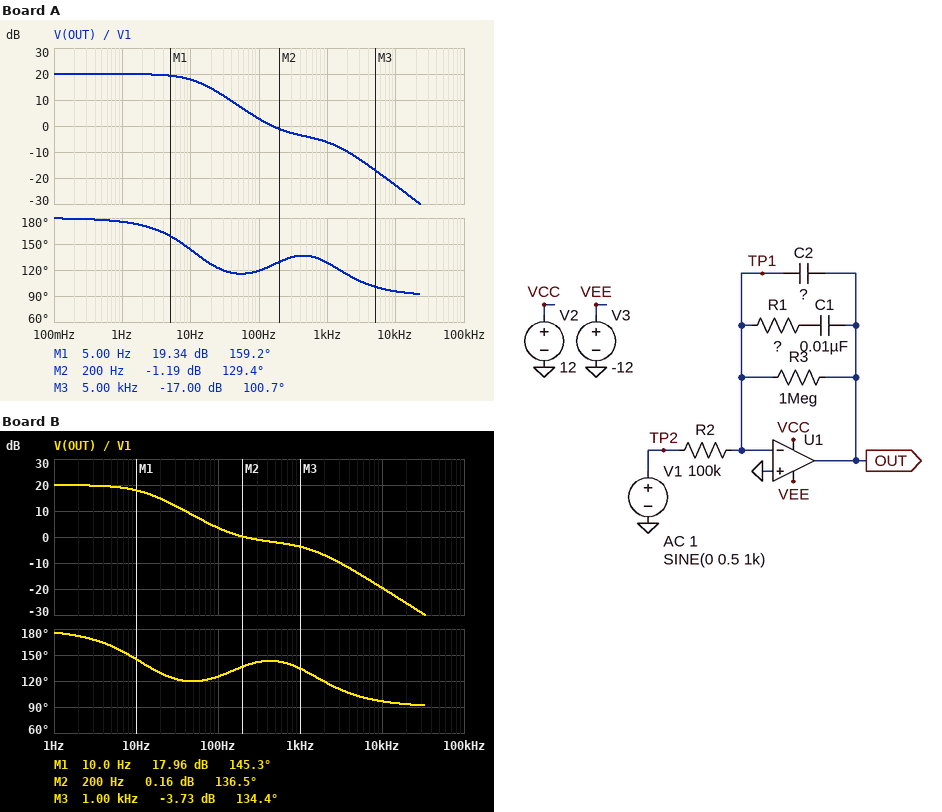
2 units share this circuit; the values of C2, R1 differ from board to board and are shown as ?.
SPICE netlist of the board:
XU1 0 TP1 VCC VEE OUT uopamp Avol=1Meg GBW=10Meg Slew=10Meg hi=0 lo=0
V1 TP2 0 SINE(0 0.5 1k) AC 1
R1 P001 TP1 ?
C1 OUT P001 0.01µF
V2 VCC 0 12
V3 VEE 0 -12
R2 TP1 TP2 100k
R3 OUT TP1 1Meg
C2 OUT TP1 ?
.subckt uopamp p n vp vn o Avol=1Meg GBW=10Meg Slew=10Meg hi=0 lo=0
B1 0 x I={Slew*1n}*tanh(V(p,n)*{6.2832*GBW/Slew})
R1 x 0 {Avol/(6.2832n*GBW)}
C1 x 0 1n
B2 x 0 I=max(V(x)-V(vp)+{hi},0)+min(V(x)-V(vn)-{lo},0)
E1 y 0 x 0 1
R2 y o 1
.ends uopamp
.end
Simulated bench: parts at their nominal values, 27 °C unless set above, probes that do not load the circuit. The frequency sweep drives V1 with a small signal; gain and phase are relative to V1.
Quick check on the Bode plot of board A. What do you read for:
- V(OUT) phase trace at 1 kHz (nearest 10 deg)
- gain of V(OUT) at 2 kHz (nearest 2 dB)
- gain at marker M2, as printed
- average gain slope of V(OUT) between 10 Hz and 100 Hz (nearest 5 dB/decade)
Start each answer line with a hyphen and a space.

- 130 deg
- -10 dB
- -1.19 dB
- -15 dB/decade
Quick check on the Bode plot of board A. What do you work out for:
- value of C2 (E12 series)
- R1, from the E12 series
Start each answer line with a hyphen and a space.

- 2.2 nF
- 82 kΩ
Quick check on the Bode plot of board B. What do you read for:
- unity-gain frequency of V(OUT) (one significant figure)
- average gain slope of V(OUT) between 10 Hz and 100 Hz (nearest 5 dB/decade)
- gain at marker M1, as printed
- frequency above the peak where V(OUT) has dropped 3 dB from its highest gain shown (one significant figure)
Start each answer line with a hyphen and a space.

- 200 Hz
- -15 dB/decade
- 17.96 dB
- 10 Hz
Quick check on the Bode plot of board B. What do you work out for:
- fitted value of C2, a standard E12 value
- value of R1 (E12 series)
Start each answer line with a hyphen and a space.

- 1.5 nF
- 100 kΩ
